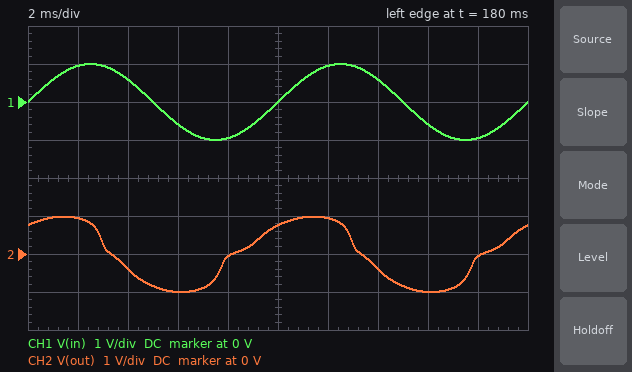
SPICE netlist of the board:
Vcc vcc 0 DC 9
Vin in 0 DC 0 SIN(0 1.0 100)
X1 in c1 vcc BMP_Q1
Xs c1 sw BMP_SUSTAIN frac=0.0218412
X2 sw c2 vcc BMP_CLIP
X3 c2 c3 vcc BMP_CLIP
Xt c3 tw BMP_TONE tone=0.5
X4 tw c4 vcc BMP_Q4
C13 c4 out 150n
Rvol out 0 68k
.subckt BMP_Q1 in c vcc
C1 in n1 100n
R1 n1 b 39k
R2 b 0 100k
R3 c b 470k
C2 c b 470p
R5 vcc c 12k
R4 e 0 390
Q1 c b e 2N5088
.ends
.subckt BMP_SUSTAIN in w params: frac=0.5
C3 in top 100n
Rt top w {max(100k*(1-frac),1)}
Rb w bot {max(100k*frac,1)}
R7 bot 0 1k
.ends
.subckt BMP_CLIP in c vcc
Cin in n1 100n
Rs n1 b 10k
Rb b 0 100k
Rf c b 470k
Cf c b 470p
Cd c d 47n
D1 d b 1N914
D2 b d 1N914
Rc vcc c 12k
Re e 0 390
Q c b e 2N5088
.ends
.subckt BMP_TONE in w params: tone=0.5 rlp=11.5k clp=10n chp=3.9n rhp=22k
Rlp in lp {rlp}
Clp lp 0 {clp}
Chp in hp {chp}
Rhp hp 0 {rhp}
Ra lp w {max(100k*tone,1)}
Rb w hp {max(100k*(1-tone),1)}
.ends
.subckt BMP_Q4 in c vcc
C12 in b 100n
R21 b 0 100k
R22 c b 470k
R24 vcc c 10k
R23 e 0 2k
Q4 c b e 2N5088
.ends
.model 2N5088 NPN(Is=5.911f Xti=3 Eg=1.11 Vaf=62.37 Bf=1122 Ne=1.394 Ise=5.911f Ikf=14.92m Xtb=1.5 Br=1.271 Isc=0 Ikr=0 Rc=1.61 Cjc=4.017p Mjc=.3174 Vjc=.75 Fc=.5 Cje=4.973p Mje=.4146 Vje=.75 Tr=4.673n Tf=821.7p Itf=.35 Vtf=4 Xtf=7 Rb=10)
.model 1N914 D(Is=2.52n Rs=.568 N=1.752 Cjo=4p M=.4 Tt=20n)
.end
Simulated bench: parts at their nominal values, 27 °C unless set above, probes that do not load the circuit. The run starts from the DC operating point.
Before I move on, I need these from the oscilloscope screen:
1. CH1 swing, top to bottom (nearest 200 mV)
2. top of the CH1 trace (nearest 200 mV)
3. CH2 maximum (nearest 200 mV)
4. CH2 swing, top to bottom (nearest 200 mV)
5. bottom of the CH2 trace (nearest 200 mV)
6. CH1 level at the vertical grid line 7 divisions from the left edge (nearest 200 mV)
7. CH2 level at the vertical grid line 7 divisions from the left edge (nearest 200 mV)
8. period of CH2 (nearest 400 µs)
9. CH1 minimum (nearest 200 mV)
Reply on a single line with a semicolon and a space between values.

2.0 V; 1.0 V; 1.0 V; 2.0 V; -1.0 V; 600 mV; -400 mV; 10.0 ms; -1.0 V
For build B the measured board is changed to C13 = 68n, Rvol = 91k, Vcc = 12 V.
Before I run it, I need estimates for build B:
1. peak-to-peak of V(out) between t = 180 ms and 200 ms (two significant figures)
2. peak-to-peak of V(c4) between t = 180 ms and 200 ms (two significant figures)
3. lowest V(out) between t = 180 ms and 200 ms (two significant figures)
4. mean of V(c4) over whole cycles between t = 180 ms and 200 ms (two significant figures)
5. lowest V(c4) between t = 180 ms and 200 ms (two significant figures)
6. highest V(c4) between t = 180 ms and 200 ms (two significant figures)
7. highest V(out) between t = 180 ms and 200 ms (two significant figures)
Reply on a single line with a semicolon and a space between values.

2.1 V; 2.4 V; -1.1 V; 8.2 V; 7.0 V; 9.3 V; 1.1 V
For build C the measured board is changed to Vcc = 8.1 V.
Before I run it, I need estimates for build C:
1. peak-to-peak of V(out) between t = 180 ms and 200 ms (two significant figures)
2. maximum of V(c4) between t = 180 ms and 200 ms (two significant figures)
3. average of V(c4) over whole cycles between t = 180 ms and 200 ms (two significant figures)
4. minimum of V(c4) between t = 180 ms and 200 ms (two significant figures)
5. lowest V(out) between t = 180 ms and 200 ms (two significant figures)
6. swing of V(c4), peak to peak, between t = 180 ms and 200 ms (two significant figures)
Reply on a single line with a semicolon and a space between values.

1.9 V; 7.0 V; 6.0 V; 5.0 V; -970 mV; 2.0 V
